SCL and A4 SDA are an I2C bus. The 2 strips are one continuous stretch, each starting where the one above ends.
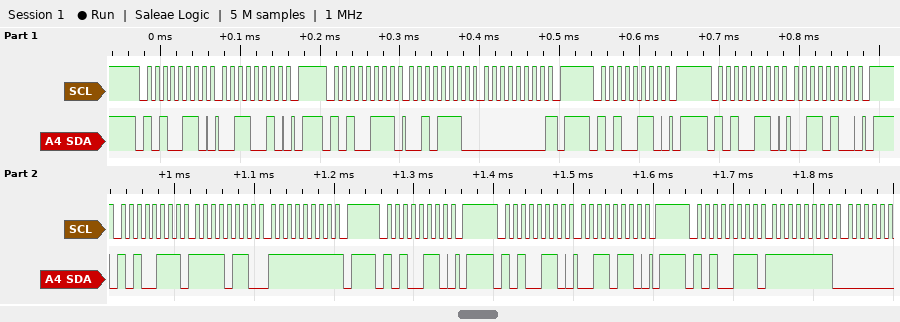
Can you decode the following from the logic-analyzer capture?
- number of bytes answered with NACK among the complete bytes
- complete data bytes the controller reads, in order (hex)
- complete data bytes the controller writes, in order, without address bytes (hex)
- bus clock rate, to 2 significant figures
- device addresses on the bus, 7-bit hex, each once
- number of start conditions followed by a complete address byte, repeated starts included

2
2E 00 F6 FF FF
32 34 36
100 kHz
0x53
8
